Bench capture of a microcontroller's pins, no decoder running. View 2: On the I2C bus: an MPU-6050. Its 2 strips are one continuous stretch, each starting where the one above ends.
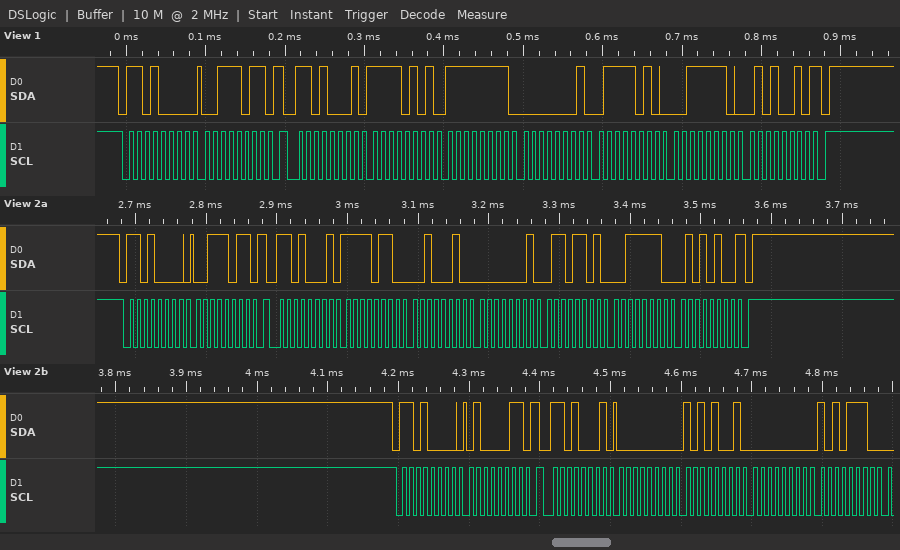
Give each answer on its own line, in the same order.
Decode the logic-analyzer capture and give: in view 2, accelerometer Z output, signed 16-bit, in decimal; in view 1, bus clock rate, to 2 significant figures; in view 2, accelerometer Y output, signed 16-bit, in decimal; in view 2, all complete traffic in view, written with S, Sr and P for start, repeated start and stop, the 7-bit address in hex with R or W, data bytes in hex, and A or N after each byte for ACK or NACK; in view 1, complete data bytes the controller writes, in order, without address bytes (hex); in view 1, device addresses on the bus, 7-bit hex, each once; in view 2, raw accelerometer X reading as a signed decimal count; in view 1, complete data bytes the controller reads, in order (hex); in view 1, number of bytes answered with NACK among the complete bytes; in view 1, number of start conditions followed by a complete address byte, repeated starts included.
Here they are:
15956
100 kHz
365
S 68W A 3B A Sr 68R A F6 A 22 A 01 A 6D A 3E A 54 N P S 68W A 43 A Sr 68R A 00 A A9 A 00 A AE A
3B
0x68
-2526
F5 FF 01 7A 3E 52
1
2
